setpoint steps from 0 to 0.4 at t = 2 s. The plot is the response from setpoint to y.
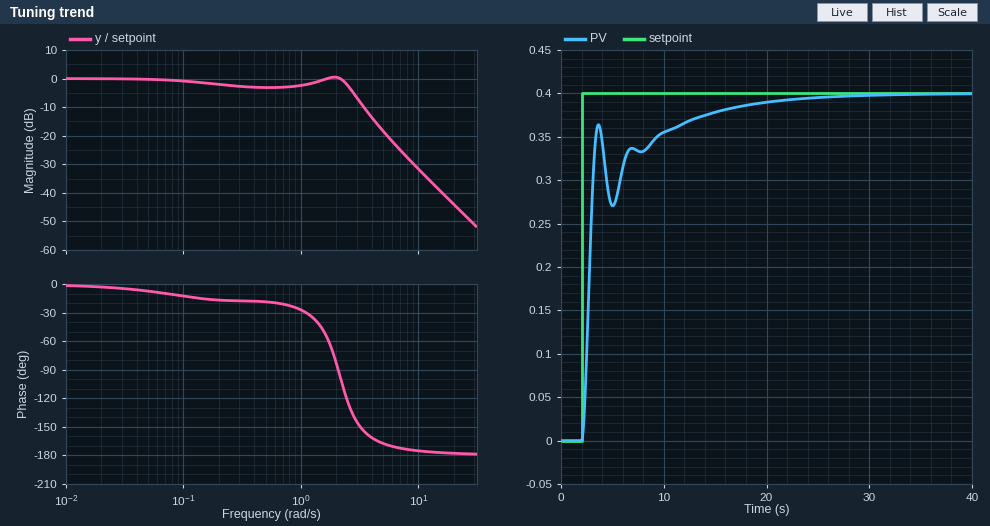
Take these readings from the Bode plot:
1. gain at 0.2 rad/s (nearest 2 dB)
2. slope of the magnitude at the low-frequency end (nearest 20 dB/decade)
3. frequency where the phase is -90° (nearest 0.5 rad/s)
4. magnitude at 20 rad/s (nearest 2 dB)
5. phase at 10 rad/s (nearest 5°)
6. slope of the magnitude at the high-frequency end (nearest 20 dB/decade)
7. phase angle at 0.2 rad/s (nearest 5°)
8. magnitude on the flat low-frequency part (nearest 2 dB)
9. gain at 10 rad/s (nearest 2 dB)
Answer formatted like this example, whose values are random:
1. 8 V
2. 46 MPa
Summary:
1. -2 dB
2. 0 dB/decade
3. 2.0 rad/s
4. -44 dB
5. -175°
6. -40 dB/decade
7. -15°
8. 0 dB
9. -32 dB
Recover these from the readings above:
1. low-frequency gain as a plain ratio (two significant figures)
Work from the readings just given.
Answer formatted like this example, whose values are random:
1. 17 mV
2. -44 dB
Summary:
1. 1.0
